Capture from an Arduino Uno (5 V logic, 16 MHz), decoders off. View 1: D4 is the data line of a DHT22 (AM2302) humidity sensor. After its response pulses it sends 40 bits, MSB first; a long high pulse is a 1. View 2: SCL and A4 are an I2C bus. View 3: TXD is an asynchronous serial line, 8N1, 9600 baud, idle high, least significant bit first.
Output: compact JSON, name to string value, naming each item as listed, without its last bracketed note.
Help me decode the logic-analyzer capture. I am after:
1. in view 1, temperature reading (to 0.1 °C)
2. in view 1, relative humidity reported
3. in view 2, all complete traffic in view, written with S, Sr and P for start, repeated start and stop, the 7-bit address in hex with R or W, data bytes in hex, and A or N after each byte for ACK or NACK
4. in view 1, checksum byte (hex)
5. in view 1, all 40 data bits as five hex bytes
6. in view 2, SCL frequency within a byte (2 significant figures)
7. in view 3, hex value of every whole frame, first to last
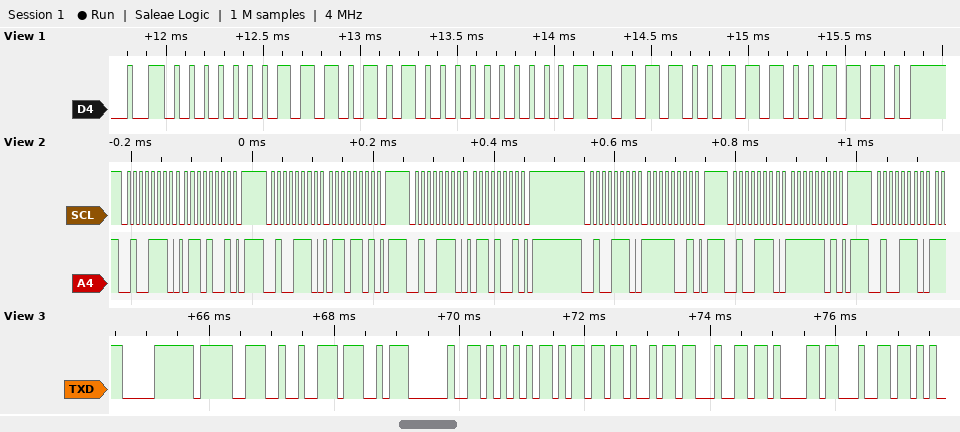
{"in view 1, temperature reading": "24.9 °C", "in view 1, relative humidity reported": "46.8 %", "in view 2, all complete traffic in view, written with S, Sr and P for start, repeated start and stop, the 7-bit address in hex with R or W, data bytes in hex, and A or N after each byte for ACK or NACK": "S 27W A 69 A P S 27W A 6D A P S 27W A 69 A P S 27W A F9 A P S 27W A FD A P S 27W A", "in view 1, checksum byte": "0xCE", "in view 1, all 40 data bits as five hex bytes": "01 D4 00 F9 CE", "in view 2, SCL frequency within a byte": "100 kHz", "in view 3, hex value of every whole frame, first to last": "F0 9F 92 A7 20 55 6D 69 64 61 64"}
